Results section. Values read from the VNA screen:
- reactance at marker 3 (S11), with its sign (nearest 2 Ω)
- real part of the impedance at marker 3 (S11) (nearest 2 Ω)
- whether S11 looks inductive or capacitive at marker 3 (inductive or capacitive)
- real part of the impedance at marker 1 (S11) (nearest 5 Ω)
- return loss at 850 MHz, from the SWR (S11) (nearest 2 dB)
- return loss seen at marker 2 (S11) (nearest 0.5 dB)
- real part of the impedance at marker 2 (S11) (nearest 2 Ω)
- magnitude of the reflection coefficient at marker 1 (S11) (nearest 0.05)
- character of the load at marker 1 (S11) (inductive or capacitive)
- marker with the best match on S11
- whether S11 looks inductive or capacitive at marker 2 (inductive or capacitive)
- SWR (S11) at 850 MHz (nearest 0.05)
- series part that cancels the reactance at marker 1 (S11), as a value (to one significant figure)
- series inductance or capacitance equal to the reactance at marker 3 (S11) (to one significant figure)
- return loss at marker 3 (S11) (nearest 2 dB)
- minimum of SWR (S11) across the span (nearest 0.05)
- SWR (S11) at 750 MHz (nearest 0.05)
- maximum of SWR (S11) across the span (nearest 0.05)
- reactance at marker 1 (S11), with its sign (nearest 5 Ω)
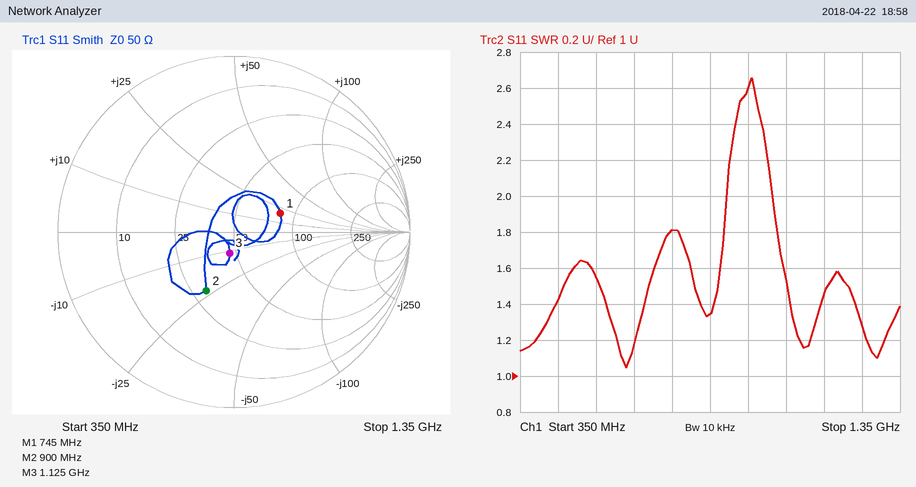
-12 Ω
46 Ω
capacitive
85 Ω
16 dB
8.5 dB
30 Ω
0.30
inductive
marker 3
capacitive
1.35
10 pF
10 pF
18 dB
1.05
1.80
2.65
+20 Ω
